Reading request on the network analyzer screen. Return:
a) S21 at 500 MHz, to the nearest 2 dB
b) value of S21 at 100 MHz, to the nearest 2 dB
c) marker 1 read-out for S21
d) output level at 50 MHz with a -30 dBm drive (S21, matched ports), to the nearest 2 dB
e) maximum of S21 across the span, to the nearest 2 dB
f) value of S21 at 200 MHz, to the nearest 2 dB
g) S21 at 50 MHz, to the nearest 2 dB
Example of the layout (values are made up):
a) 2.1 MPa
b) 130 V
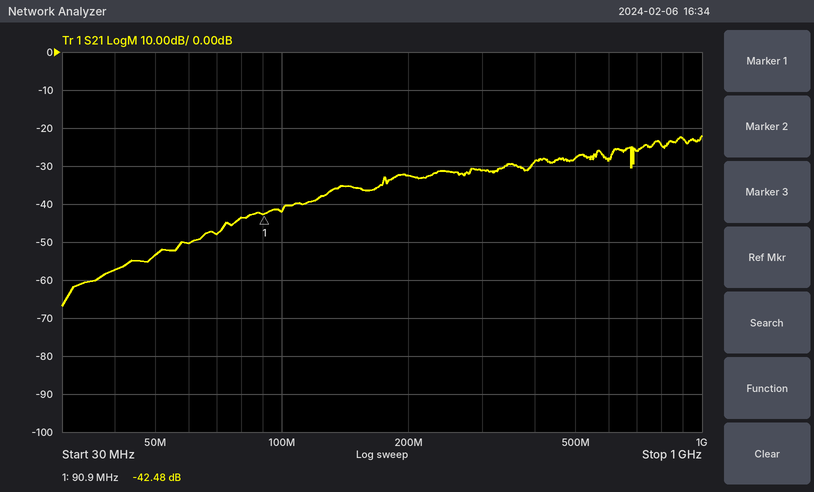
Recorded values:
a) -28 dB
b) -42 dB
c) -42.48 dB
d) -84 dBm
e) -22 dB
f) -32 dB
g) -54 dB
